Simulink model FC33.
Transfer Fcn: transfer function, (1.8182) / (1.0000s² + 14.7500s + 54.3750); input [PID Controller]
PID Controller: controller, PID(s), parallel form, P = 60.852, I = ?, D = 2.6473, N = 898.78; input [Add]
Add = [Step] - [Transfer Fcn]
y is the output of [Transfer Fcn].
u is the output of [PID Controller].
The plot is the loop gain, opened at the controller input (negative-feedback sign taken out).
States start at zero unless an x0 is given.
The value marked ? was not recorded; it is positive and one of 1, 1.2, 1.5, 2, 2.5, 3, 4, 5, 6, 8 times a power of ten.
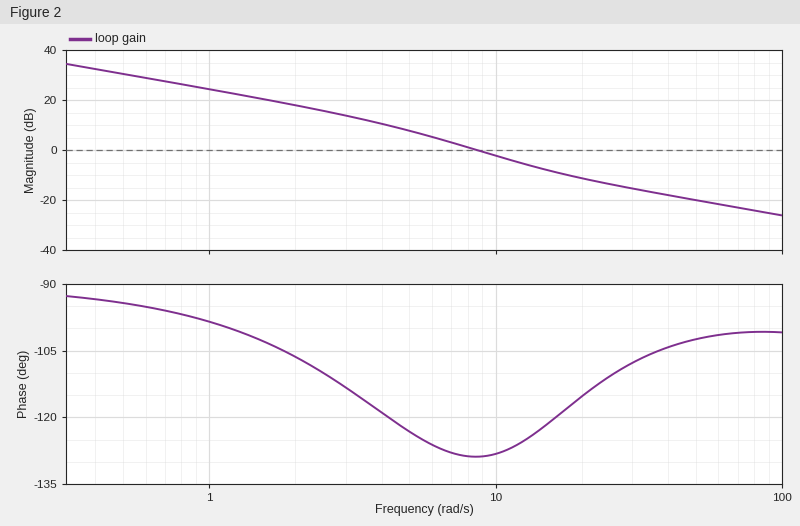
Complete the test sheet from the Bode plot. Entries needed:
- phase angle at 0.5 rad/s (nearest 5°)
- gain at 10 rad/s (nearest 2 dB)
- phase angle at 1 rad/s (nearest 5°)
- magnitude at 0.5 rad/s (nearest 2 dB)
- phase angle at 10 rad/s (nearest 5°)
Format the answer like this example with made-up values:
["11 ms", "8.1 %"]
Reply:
["-95°", "-2 dB", "-100°", "30 dB", "-130°"]
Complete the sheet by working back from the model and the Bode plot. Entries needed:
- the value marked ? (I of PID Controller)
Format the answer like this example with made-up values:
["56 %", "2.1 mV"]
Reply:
["500"]
